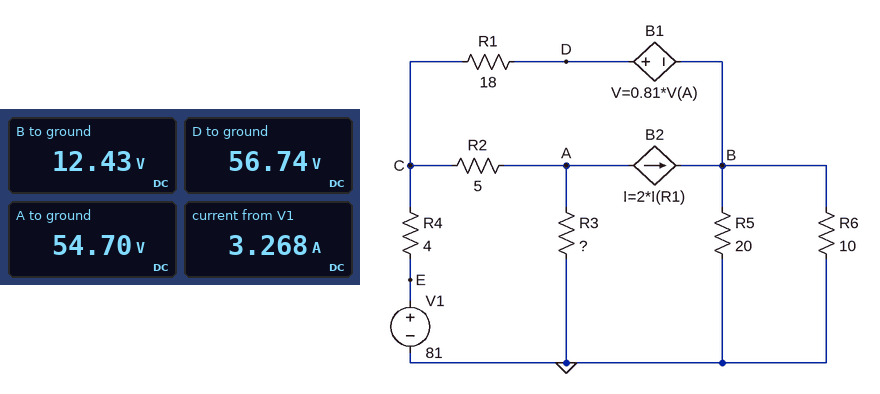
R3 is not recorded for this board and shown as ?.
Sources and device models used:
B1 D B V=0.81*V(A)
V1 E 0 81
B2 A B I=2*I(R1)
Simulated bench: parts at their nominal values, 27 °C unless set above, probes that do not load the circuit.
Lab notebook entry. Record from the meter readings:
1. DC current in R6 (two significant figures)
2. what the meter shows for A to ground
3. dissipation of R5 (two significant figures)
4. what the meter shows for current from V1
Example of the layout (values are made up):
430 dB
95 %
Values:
1.2 A
54.70 V
7.7 W
3.268 A
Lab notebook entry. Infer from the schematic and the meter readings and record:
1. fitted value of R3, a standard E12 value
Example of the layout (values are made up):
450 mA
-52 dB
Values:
39 Ω
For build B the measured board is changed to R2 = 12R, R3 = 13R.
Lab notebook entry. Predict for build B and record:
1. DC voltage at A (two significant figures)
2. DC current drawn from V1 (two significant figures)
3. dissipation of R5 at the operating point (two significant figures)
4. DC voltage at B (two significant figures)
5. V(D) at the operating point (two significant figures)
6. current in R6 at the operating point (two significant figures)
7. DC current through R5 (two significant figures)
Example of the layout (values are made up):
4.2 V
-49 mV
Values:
16 V
5.0 A
32 W
25 V
38 V
2.5 A
1.3 A
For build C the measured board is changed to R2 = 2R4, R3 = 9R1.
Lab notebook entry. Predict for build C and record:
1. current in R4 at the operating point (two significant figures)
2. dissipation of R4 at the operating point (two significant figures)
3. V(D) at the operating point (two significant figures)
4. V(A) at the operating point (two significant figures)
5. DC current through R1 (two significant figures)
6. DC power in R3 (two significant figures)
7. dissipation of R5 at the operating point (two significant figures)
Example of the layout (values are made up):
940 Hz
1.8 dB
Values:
6.3 A
160 W
45 V
42 V
570 mA
190 W
6.6 W
